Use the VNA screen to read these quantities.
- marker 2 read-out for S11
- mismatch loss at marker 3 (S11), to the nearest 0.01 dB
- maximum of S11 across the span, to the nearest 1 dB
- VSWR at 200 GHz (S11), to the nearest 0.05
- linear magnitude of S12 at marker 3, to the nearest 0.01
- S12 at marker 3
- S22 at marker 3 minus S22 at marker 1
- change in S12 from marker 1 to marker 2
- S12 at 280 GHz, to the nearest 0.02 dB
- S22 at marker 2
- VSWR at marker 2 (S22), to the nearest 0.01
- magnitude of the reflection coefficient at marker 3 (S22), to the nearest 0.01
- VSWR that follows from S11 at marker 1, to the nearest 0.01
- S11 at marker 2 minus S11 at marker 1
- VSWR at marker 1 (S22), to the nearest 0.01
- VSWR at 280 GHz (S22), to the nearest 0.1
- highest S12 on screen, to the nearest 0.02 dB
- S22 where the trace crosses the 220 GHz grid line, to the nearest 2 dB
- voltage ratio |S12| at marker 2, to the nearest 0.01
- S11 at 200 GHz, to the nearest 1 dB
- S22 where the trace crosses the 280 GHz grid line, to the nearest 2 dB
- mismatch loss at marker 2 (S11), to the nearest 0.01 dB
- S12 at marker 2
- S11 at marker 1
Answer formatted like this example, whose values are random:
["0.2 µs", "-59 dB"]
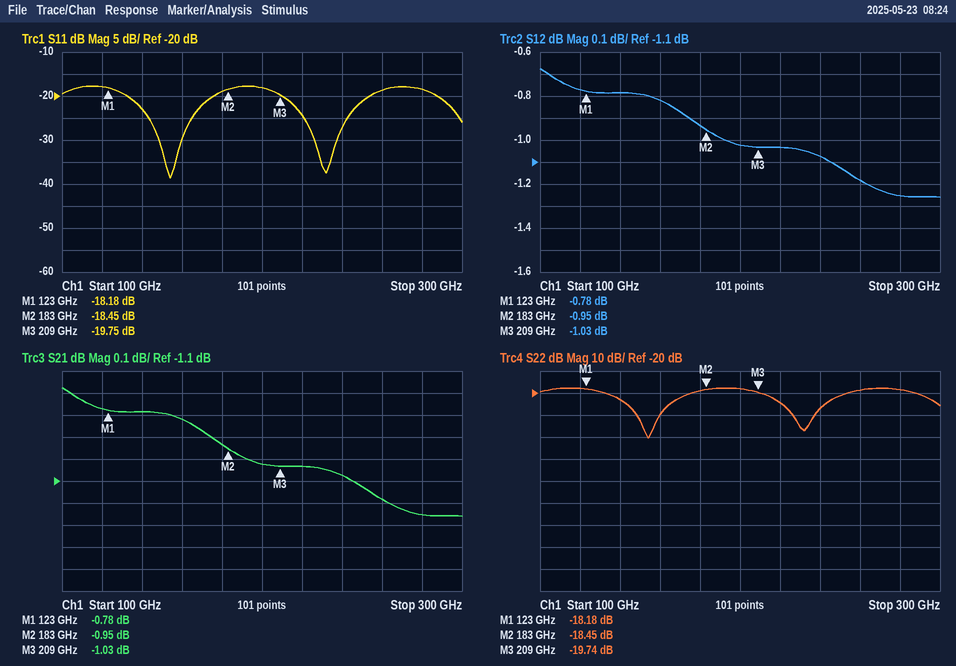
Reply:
["-18.45 dB", "0.05 dB", "-18 dB", "1.30", "0.89", "-1.03 dB", "-1.56 dB", "-0.17 dB", "-1.26 dB", "-18.45 dB", "1.27", "0.10", "1.28", "-0.27 dB", "1.28", "1.3", "-0.68 dB", "-24 dB", "0.90", "-18 dB", "-18 dB", "0.06 dB", "-0.95 dB", "-18.18 dB"]
